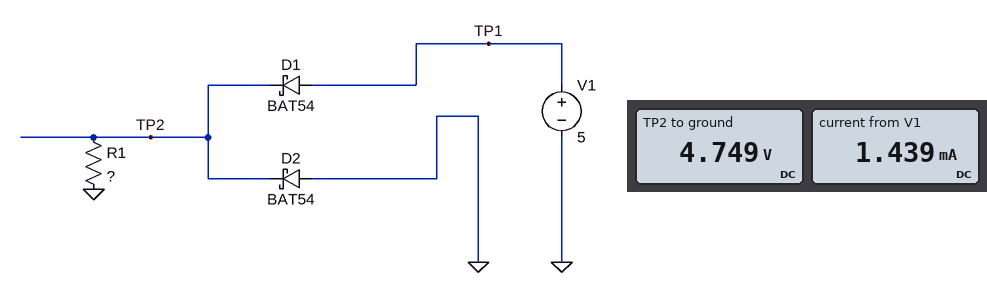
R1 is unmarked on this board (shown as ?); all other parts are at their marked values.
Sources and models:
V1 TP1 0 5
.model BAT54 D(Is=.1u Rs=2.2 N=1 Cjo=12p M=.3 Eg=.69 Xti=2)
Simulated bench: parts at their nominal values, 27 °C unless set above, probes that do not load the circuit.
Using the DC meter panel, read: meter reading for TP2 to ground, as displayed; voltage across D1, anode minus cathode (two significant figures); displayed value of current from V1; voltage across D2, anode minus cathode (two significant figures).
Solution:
4.749 V
250 mV
1.439 mA
-4.7 V
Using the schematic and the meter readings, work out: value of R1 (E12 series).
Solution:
3.3 kΩ
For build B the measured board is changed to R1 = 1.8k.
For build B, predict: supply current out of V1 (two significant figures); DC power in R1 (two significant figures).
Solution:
2.6 mA
12 mW
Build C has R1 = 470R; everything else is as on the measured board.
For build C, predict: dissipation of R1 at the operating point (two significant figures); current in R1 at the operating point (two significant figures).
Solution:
47 mW
10 mA
